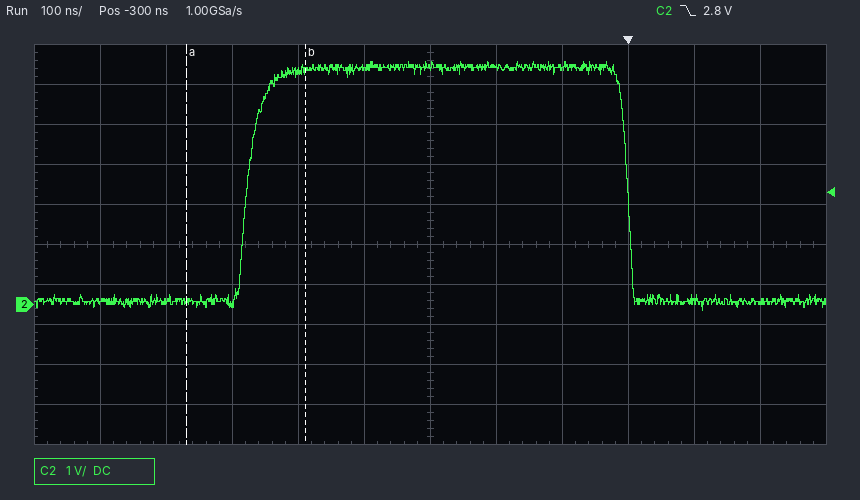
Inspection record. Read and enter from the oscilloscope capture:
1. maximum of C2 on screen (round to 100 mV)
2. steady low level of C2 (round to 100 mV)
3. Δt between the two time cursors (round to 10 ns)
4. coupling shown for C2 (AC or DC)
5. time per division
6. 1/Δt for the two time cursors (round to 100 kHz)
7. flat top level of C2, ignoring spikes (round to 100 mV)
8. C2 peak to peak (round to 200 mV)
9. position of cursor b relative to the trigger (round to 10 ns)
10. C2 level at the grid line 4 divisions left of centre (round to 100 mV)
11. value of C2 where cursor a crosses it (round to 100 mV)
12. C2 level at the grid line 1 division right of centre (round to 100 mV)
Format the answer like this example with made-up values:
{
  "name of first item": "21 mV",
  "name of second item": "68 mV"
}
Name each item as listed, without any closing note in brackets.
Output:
{
  "maximum of C2 on screen": "6.1 V",
  "steady low level of C2": "100 mV",
  "Δt between the two time cursors": "180 ns",
  "coupling shown for C2": "DC",
  "time per division": "100 ns",
  "1/Δt for the two time cursors": "5.6 MHz",
  "flat top level of C2, ignoring spikes": "5.9 V",
  "C2 peak to peak": "6.2 V",
  "position of cursor b relative to the trigger": "-490 ns",
  "C2 level at the grid line 4 divisions left of centre": "100 mV",
  "value of C2 where cursor a crosses it": "100 mV",
  "C2 level at the grid line 1 division right of centre": "5.9 V"
}
